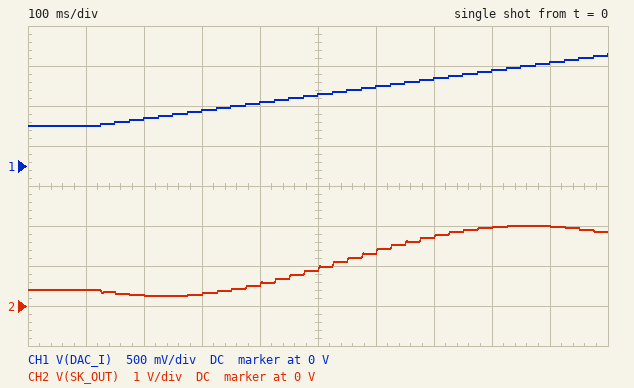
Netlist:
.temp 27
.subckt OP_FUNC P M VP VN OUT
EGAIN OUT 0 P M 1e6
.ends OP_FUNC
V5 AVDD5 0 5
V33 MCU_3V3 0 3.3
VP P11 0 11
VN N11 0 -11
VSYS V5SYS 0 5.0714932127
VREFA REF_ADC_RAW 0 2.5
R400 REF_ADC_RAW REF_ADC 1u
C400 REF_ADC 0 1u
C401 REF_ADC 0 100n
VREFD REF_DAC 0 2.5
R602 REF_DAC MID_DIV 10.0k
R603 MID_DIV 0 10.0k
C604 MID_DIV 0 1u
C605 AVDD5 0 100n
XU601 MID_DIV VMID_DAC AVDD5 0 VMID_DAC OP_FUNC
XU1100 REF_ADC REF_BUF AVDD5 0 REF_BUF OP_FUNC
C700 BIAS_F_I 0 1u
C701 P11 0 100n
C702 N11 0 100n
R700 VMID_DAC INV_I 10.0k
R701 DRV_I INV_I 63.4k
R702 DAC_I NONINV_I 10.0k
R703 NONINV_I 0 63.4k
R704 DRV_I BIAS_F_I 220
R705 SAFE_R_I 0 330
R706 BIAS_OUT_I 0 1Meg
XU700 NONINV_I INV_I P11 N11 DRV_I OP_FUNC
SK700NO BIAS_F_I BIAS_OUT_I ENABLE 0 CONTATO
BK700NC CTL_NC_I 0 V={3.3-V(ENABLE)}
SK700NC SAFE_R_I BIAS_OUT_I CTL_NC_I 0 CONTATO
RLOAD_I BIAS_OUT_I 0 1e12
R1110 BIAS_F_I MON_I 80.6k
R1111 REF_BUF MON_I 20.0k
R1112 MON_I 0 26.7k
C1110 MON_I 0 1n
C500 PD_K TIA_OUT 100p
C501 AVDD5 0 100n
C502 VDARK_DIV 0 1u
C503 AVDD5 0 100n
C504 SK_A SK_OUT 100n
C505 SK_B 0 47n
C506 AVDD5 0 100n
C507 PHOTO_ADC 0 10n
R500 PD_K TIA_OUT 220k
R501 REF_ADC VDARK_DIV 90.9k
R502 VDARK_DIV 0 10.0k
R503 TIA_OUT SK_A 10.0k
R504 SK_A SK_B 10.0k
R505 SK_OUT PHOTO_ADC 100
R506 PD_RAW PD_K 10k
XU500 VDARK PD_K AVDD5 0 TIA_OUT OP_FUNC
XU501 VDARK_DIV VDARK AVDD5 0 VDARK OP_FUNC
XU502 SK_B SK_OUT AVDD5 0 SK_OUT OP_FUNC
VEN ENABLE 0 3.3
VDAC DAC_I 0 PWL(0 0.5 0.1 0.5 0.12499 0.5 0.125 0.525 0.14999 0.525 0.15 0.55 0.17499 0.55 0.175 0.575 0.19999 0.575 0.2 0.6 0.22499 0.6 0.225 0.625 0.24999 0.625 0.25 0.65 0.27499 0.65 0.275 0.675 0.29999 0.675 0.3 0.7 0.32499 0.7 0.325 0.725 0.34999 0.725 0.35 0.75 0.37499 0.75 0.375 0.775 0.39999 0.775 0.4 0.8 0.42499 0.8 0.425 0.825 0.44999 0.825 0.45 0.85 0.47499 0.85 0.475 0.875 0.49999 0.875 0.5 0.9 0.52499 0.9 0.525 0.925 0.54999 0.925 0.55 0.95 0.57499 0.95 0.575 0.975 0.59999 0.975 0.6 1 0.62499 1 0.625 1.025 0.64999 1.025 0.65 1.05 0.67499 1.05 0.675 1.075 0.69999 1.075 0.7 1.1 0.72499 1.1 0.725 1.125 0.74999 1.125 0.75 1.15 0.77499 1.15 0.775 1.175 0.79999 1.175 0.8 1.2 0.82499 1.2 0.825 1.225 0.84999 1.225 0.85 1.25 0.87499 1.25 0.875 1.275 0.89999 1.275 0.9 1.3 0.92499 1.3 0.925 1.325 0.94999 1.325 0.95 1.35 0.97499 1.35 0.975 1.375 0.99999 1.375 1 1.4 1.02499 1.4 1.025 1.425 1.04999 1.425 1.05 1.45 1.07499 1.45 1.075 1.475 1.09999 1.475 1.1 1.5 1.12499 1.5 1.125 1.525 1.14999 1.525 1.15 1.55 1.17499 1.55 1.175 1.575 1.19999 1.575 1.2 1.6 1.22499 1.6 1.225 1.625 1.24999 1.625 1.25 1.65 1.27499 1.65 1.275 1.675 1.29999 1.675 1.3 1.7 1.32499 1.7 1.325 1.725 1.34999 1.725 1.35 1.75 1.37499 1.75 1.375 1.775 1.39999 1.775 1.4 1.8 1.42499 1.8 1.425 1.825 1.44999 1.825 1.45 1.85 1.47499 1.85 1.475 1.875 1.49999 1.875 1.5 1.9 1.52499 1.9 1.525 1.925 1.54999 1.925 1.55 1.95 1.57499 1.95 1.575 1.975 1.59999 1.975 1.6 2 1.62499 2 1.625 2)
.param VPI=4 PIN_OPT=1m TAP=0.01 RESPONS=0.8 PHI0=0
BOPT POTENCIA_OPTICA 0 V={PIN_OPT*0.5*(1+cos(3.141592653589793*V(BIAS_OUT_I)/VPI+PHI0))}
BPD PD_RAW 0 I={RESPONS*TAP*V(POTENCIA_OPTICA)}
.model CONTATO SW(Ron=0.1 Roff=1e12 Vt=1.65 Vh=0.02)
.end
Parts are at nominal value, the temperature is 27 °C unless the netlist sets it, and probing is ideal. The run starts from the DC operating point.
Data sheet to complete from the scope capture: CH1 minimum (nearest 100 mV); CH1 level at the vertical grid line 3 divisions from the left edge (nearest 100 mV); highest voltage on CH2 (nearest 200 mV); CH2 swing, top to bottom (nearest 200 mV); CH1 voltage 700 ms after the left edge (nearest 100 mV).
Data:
500 mV
700 mV
2.0 V
1.8 V
1.1 V
